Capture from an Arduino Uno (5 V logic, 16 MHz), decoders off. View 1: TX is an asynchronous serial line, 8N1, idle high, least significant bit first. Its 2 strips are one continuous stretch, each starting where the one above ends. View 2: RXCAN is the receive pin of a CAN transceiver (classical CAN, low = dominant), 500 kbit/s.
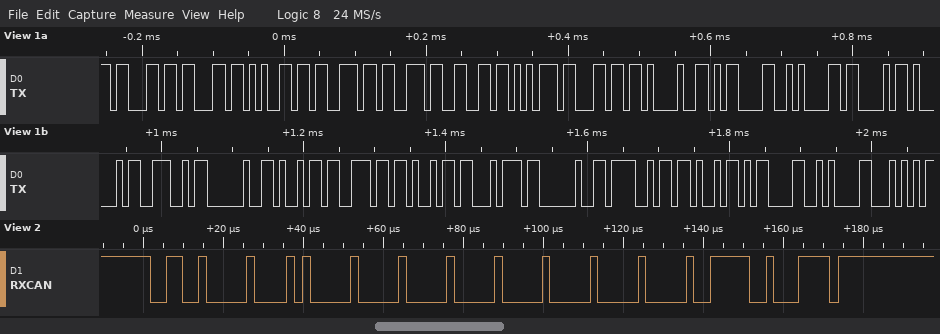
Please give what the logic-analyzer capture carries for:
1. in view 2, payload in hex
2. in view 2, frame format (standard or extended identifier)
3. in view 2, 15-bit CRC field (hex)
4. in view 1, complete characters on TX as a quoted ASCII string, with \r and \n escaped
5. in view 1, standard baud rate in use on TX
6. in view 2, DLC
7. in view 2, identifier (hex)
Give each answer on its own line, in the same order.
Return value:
00 00 00 00 00
standard
0x1F47
"ccessful!\r\nCAN init OK\r\nT"
115200 baud
5
0x320
